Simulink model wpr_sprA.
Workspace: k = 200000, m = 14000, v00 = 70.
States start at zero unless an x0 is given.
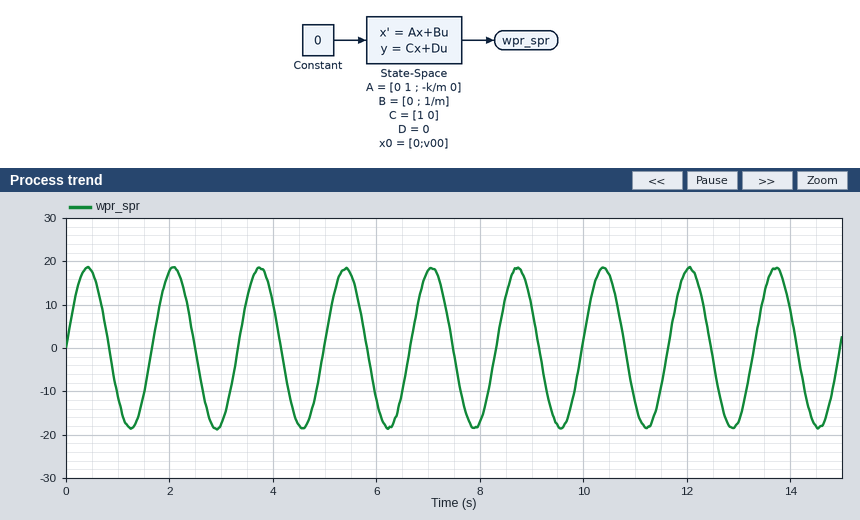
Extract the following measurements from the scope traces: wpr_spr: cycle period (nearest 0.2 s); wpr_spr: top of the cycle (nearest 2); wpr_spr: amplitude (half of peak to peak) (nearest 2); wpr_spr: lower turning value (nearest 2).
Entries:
1.6 s
18
18
-18
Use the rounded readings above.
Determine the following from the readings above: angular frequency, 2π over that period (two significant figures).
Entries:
3.9 rad/s
